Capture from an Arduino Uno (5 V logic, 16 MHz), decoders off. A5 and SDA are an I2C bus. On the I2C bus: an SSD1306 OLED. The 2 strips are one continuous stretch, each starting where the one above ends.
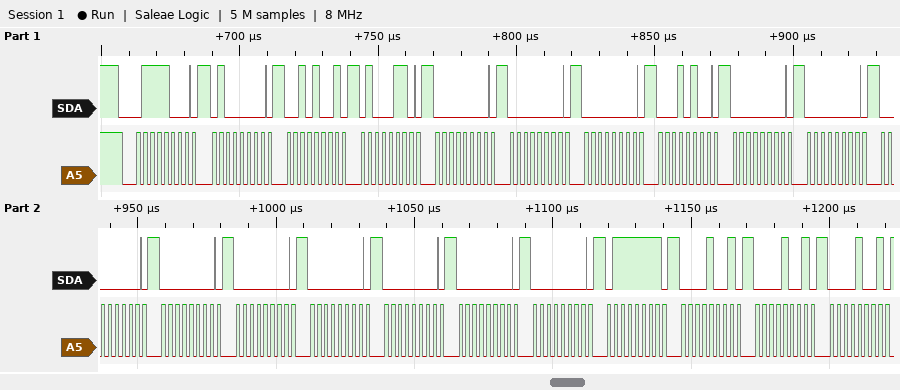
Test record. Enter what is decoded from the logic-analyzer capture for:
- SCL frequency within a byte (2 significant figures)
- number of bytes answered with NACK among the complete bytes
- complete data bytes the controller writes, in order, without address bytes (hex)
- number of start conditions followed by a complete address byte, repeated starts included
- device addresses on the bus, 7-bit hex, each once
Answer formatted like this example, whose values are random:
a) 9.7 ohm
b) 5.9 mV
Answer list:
a) 400 kHz
b) 0
c) 40 29 46 00 00 00 14 00 00 00 00 00 00 00 00 00 7F 09 09 09
d) 1
e) 0x3C
